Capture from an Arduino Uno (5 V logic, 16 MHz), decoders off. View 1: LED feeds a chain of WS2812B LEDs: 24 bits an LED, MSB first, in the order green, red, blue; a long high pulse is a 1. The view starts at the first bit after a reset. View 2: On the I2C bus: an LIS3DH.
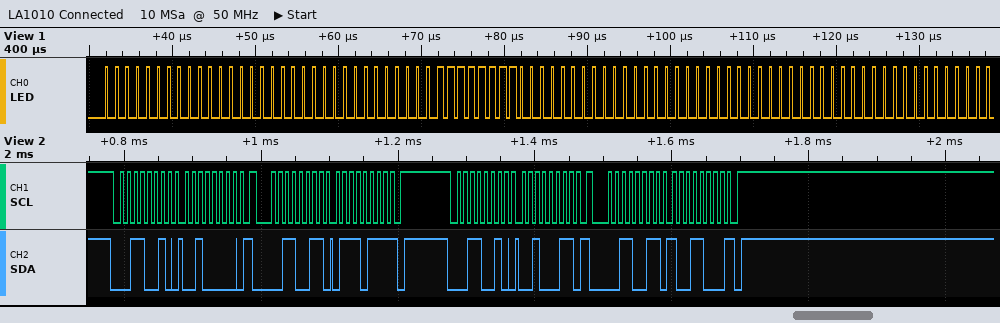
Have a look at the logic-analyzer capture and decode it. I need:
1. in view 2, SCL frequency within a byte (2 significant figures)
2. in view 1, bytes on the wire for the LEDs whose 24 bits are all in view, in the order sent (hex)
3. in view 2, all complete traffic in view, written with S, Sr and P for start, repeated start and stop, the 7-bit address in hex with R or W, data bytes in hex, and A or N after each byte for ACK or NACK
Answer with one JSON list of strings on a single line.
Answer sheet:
["100 kHz", "00 00 00 00 FF 00 00 00 00", "S 19W A 20 A Sr 19R A 77 N P S 19W A 23 A Sr 19R A 98 N P"]
